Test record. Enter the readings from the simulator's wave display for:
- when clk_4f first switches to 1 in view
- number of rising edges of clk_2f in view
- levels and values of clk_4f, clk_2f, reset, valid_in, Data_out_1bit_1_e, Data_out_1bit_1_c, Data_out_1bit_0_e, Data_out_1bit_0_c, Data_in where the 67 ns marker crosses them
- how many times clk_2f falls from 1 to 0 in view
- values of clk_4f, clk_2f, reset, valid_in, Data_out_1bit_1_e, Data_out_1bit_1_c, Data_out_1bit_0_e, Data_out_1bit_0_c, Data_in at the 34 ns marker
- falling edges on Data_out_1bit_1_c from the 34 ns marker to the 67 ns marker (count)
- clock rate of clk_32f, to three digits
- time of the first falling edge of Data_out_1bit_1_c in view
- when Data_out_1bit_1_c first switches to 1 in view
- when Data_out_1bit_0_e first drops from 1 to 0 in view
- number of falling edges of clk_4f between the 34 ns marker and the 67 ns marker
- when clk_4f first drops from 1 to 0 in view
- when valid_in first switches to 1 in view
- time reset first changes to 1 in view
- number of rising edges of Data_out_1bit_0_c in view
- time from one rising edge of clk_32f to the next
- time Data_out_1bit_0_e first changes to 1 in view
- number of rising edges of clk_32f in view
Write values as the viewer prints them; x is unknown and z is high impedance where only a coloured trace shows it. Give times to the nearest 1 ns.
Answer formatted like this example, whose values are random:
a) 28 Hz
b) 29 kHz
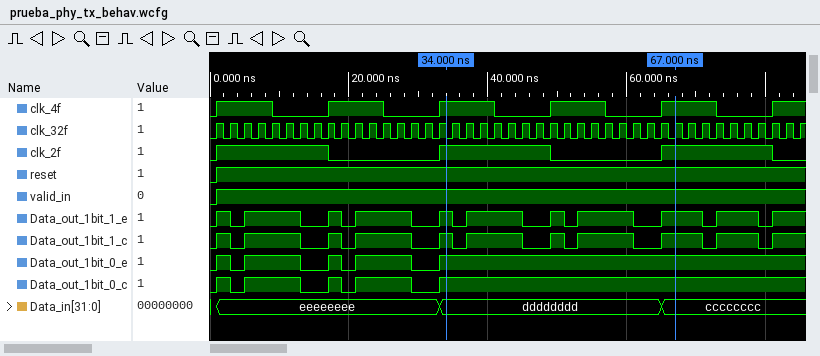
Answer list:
a) 1 ns
b) 3
c) clk_4f=1, clk_2f=1, reset=1, valid_in=1, Data_out_1bit_1_e=1, Data_out_1bit_1_c=1, Data_out_1bit_0_e=1, Data_out_1bit_0_c=1, Data_in=cccccccc
d) 3
e) clk_4f=1, clk_2f=1, reset=1, valid_in=1, Data_out_1bit_1_e=1, Data_out_1bit_1_c=1, Data_out_1bit_0_e=1, Data_out_1bit_0_c=1, Data_in=dddddddd
f) 4
g) 500 MHz
h) 3 ns
i) 1 ns
j) 3 ns
k) 2
l) 9 ns
m) 1 ns
n) 1 ns
o) 5
p) 2 ns
q) 1 ns
r) 43
